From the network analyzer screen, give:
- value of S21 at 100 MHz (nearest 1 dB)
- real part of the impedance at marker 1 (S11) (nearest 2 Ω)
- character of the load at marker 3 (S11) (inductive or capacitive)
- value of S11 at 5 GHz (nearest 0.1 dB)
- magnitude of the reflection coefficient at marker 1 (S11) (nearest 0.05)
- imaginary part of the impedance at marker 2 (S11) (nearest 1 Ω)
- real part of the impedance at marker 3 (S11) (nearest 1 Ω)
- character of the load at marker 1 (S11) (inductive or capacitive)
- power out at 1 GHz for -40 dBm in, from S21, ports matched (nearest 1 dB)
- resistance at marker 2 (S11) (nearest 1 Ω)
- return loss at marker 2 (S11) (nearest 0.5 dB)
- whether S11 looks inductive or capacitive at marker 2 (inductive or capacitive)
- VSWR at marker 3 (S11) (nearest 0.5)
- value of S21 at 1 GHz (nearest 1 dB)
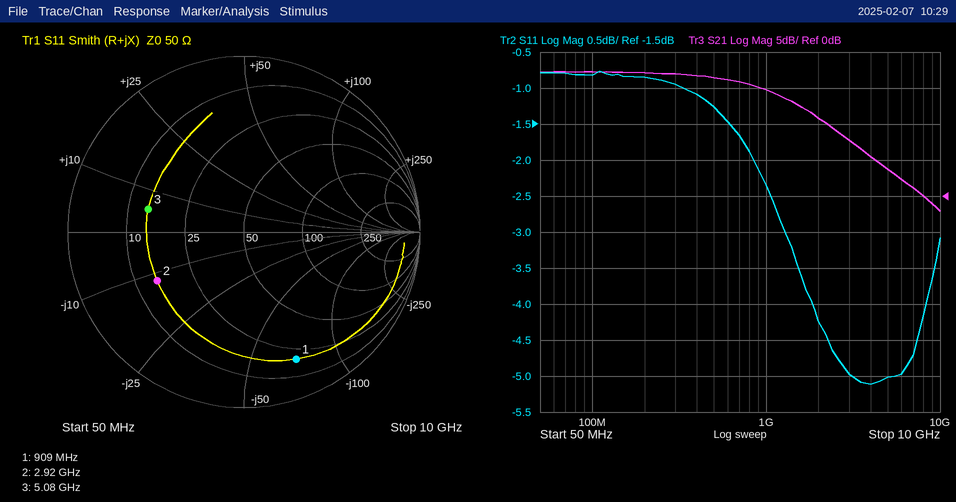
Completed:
17 dB
20 Ω
inductive
-5.0 dB
0.80
-12 Ω
14 Ω
capacitive
-25 dBm
15 Ω
5.0 dB
capacitive
3.5
15 dB
